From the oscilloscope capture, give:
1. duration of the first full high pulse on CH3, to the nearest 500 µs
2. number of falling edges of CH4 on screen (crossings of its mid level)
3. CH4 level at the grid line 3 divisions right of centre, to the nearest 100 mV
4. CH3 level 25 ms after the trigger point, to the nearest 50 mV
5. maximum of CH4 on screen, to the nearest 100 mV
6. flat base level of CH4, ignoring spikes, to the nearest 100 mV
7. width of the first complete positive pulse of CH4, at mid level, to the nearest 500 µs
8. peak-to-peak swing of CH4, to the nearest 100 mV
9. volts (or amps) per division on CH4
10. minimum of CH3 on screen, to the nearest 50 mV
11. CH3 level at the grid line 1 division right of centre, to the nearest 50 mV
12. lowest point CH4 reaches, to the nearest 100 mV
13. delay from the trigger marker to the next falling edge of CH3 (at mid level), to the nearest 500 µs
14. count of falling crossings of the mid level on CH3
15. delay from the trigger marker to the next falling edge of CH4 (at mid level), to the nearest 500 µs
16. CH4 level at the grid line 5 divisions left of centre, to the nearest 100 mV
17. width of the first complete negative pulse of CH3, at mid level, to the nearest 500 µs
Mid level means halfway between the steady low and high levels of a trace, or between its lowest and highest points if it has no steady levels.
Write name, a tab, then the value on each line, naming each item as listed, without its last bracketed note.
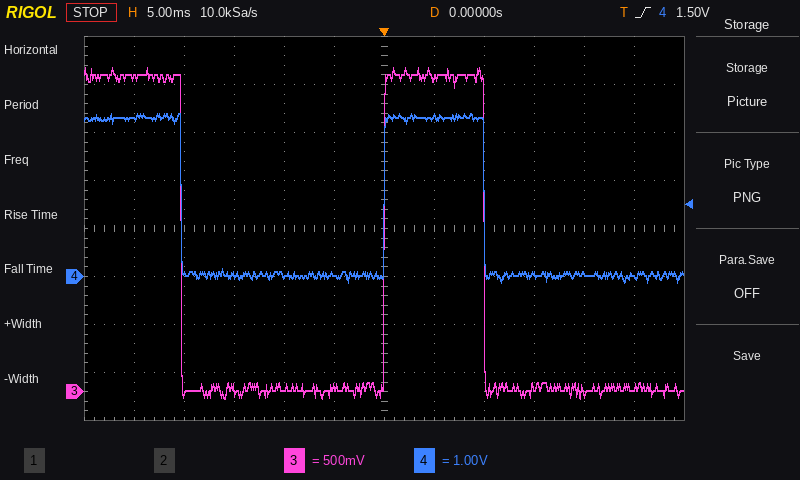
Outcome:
duration of the first full high pulse on CH3, to the nearest 500 µs	10.0 ms
number of falling edges of CH4 on screen	2
CH4 level at the grid line 3 divisions right of centre, to the nearest 100 mV	0.0 V
CH3 level 25 ms after the trigger point, to the nearest 50 mV	50 mV
maximum of CH4 on screen, to the nearest 100 mV	3.4 V
flat base level of CH4, ignoring spikes, to the nearest 100 mV	0.0 V
width of the first complete positive pulse of CH4, at mid level, to the nearest 500 µs	10.0 ms
peak-to-peak swing of CH4, to the nearest 100 mV	3.5 V
volts (or amps) per division on CH4	1 V
minimum of CH3 on screen, to the nearest 50 mV	-50 mV
CH3 level at the grid line 1 division right of centre, to the nearest 50 mV	3.25 V
lowest point CH4 reaches, to the nearest 100 mV	-100 mV
delay from the trigger marker to the next falling edge of CH3 (at mid level), to the nearest 500 µs	10.0 ms
count of falling crossings of the mid level on CH3	2
delay from the trigger marker to the next falling edge of CH4 (at mid level), to the nearest 500 µs	10.0 ms
CH4 level at the grid line 5 divisions left of centre, to the nearest 100 mV	3.3 V
width of the first complete negative pulse of CH3, at mid level, to the nearest 500 µs	20.5 ms
